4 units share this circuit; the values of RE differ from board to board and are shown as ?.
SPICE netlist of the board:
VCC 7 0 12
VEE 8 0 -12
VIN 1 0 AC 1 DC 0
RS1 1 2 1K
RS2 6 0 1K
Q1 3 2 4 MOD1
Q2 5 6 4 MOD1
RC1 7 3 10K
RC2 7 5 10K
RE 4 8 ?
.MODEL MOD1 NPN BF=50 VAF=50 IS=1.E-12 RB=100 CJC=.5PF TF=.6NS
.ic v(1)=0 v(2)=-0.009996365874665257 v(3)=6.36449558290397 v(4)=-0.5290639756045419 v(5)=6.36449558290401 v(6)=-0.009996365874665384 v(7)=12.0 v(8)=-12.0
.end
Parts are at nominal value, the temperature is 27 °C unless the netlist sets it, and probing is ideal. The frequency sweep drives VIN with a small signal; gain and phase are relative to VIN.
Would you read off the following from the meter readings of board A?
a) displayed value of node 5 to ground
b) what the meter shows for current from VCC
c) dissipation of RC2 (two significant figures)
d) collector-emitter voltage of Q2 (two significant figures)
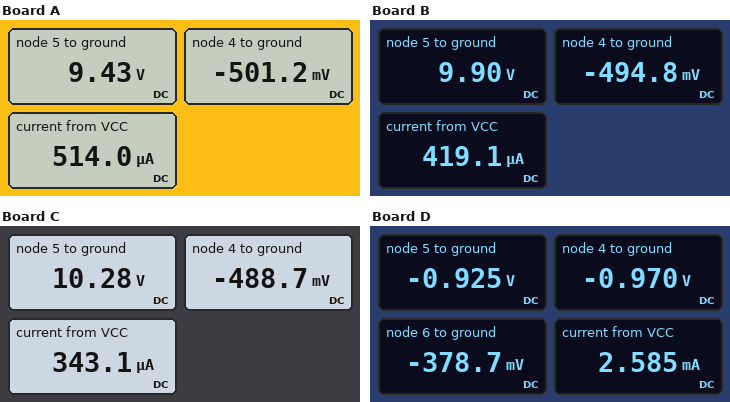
9.43 V
514.0 µA
660 µW
9.9 V
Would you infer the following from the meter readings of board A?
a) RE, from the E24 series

22 kΩ
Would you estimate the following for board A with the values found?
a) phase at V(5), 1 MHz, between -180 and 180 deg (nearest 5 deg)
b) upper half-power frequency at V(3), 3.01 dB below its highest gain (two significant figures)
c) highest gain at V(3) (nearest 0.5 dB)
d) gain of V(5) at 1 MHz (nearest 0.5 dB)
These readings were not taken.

-10 deg
6.2 MHz
32.0 dB
32.0 dB
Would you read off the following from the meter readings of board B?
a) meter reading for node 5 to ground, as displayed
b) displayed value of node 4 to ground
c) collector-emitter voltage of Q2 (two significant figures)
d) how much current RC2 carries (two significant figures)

9.90 V
-494.8 mV
10 V
210 µA
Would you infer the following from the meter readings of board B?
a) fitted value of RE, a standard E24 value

27 kΩ
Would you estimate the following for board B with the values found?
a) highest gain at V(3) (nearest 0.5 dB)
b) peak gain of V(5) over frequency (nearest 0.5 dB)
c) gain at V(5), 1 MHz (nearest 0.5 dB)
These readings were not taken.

30.5 dB
30.5 dB
30.5 dB
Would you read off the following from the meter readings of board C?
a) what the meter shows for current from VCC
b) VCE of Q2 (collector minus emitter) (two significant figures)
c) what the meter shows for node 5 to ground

343.1 µA
11 V
10.28 V
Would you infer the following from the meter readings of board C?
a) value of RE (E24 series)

33 kΩ
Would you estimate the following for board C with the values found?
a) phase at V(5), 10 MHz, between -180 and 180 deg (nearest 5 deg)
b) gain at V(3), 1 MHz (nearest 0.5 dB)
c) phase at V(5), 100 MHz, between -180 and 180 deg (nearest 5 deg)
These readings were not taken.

-50 deg
29.0 dB
-95 deg
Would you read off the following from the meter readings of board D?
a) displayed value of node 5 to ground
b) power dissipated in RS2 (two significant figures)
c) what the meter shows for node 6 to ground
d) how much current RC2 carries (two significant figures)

-0.925 V
140 µW
-378.7 mV
1.3 mA
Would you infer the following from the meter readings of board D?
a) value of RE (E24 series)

3.3 kΩ
